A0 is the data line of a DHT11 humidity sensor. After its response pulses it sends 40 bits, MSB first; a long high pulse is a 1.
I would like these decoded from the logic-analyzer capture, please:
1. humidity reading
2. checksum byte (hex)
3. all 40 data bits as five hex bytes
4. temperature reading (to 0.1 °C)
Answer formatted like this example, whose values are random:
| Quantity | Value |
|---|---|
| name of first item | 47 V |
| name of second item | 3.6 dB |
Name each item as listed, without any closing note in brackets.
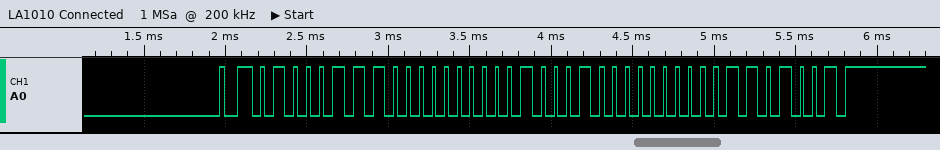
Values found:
| Quantity | Value |
|---|---|
| humidity reading | 71 % |
| checksum byte | 0x69 |
| all 40 data bits as five hex bytes | 47 00 22 00 69 |
| temperature reading | 34.0 °C |
